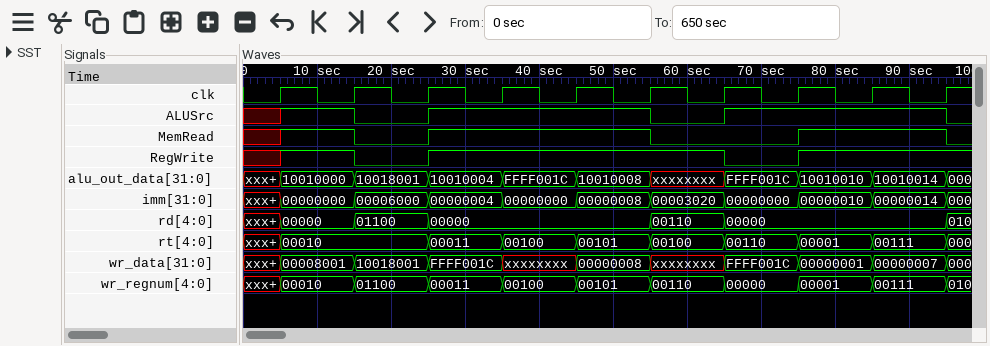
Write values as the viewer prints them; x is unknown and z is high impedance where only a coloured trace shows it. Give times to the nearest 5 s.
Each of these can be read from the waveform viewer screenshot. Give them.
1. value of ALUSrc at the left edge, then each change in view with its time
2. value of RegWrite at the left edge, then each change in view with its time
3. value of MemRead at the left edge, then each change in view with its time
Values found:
x, 1 at 5 s, 0 at 15 s, 1 at 25 s, 0 at 55 s, 1 at 65 s, 0 at 95 s
x, 1 at 5 s, 0 at 15 s, 1 at 25 s, 0 at 65 s, 1 at 75 s
x, 1 at 5 s, 0 at 15 s, 1 at 25 s, 0 at 55 s, 1 at 75 s, 0 at 95 s
